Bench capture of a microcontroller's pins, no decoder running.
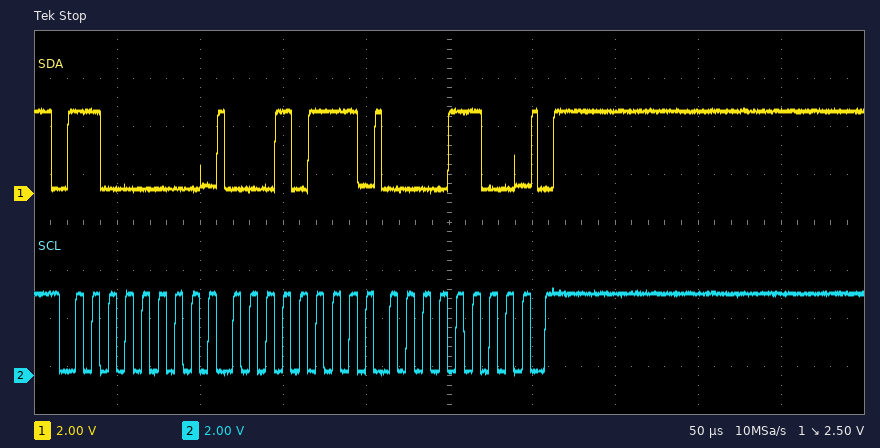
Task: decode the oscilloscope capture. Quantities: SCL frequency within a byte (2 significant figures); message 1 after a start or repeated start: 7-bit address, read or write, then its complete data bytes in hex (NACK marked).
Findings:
100 kHz
0x60 write: 17 0C
